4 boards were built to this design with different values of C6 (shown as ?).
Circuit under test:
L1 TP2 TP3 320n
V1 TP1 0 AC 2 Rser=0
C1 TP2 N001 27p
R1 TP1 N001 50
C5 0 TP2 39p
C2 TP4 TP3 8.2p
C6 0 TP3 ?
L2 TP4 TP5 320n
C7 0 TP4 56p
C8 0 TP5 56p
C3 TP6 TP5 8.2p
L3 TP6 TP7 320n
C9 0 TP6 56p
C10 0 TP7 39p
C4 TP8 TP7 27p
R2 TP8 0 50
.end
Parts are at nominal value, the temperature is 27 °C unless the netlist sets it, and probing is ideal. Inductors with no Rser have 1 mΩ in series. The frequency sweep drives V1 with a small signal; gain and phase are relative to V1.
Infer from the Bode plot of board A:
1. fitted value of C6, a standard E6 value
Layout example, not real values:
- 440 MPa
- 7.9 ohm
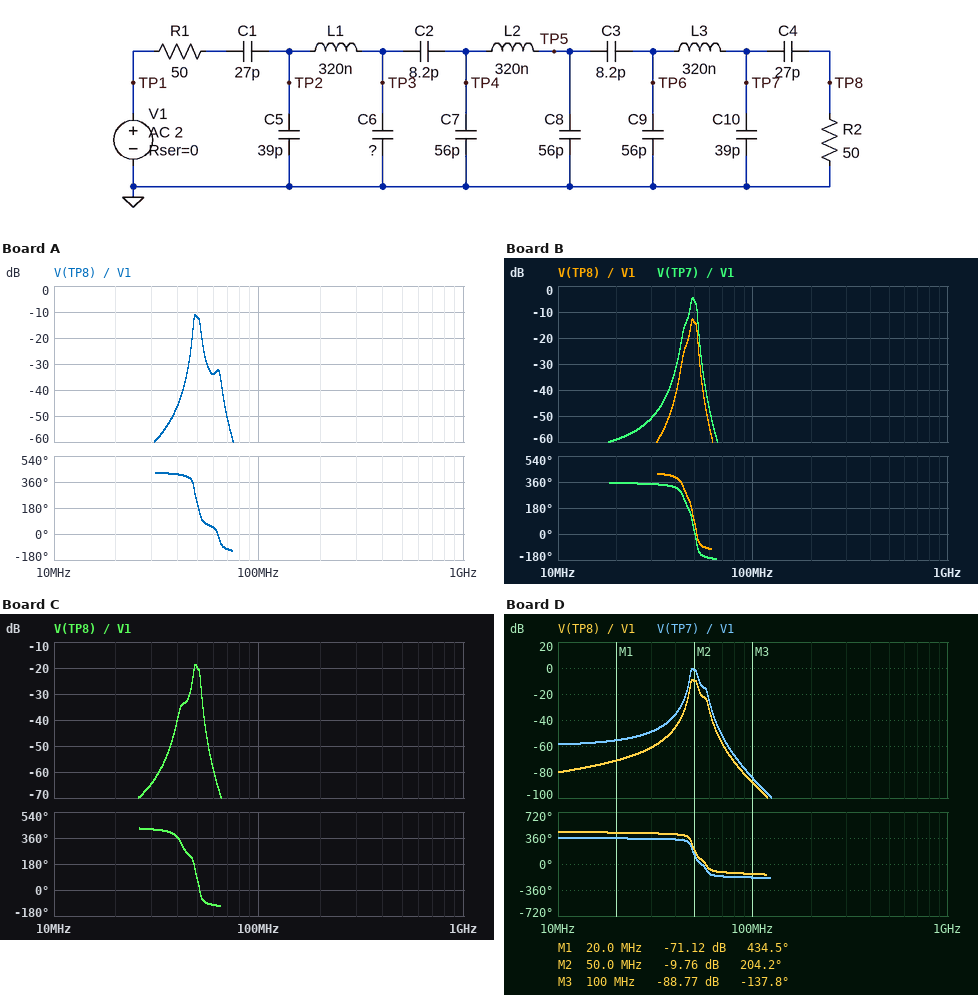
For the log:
- 22 pF
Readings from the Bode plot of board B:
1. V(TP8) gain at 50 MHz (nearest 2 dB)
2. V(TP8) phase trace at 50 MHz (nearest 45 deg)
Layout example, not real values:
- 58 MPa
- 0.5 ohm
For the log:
- -14 dB
- 90 deg
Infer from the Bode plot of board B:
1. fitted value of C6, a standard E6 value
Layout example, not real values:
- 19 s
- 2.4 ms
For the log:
- 100 pF
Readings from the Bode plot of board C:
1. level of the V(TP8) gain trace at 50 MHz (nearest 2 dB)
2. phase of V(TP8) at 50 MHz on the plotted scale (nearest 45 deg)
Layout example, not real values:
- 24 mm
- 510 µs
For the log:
- -20 dB
- 90 deg
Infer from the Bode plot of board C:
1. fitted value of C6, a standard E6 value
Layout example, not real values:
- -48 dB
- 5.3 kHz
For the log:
- 150 pF
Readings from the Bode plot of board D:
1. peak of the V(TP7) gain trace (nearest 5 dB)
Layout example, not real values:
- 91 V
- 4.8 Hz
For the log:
- 0 dB
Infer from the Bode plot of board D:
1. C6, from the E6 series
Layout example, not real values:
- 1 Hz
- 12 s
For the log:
- 33 pF
